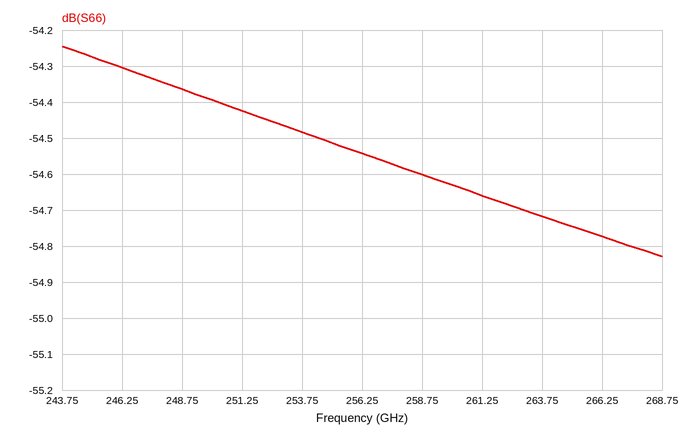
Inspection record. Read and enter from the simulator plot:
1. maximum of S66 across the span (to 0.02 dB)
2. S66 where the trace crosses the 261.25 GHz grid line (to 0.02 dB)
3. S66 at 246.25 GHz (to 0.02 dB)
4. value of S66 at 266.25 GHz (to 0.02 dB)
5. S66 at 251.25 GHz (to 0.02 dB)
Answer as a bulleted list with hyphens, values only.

- -54.24 dB
- -54.66 dB
- -54.30 dB
- -54.78 dB
- -54.42 dB
